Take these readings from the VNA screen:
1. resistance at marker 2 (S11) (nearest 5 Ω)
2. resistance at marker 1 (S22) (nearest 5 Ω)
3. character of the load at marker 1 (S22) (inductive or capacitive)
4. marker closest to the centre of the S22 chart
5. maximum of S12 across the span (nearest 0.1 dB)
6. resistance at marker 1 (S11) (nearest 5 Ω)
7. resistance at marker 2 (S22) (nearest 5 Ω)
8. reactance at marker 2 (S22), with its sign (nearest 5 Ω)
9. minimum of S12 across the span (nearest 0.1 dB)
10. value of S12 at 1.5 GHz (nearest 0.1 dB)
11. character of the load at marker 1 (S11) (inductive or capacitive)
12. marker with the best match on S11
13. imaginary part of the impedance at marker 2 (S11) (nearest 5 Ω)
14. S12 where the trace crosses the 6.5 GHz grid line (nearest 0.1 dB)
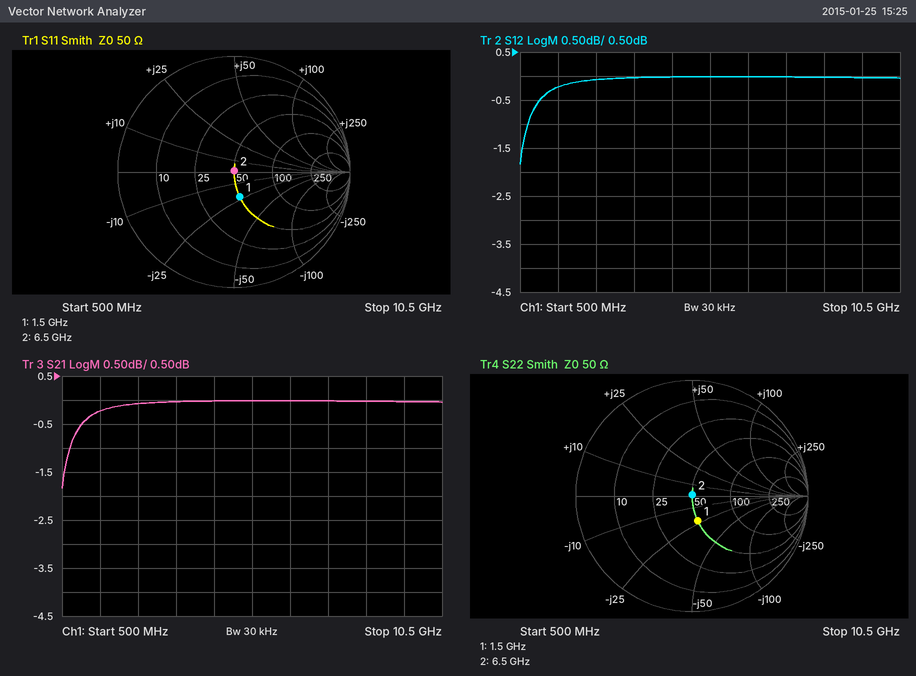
50 Ω
50 Ω
capacitive
marker 2
0.0 dB
50 Ω
50 Ω
0 Ω
-1.8 dB
-0.2 dB
capacitive
marker 2
0 Ω
0.0 dB
